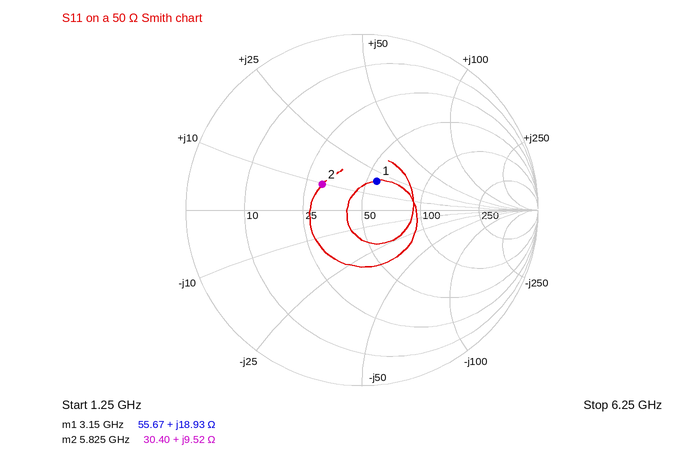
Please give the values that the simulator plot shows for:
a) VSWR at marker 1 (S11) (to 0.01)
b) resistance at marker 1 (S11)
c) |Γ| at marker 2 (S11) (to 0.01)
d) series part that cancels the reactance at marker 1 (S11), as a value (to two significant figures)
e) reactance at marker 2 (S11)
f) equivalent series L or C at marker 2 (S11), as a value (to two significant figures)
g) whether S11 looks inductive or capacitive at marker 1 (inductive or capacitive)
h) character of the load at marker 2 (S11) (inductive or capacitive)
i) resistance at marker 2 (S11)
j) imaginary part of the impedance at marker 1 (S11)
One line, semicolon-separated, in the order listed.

1.45; 55.67 Ω; 0.27; 2.7 pF; +9.52 Ω; 260 pH; inductive; inductive; 30.40 Ω; +18.93 Ω
